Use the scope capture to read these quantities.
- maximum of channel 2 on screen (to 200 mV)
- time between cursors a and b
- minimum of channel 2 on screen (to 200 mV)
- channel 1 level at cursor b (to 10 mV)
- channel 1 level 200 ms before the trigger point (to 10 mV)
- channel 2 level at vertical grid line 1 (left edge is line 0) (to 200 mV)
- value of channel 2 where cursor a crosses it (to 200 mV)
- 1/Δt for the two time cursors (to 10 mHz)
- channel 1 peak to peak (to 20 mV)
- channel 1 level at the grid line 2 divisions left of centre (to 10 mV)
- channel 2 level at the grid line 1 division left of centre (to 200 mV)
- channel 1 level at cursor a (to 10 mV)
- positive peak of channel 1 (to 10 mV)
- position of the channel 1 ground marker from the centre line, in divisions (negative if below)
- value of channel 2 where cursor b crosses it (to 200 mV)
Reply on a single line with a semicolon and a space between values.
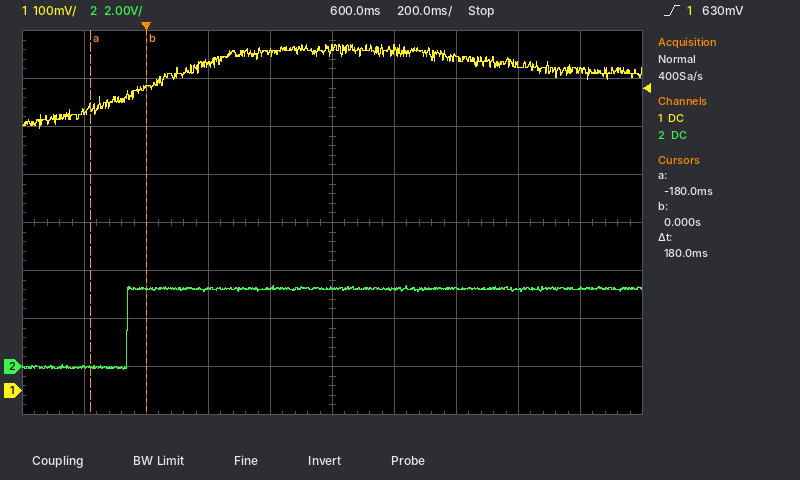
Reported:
3.4 V; 180 ms; -200 mV; 630 mV; 580 mV; 0.0 V; 0.0 V; 5.56 Hz; 180 mV; 680 mV; 3.2 V; 590 mV; 720 mV; -3.5 div; 3.2 V
